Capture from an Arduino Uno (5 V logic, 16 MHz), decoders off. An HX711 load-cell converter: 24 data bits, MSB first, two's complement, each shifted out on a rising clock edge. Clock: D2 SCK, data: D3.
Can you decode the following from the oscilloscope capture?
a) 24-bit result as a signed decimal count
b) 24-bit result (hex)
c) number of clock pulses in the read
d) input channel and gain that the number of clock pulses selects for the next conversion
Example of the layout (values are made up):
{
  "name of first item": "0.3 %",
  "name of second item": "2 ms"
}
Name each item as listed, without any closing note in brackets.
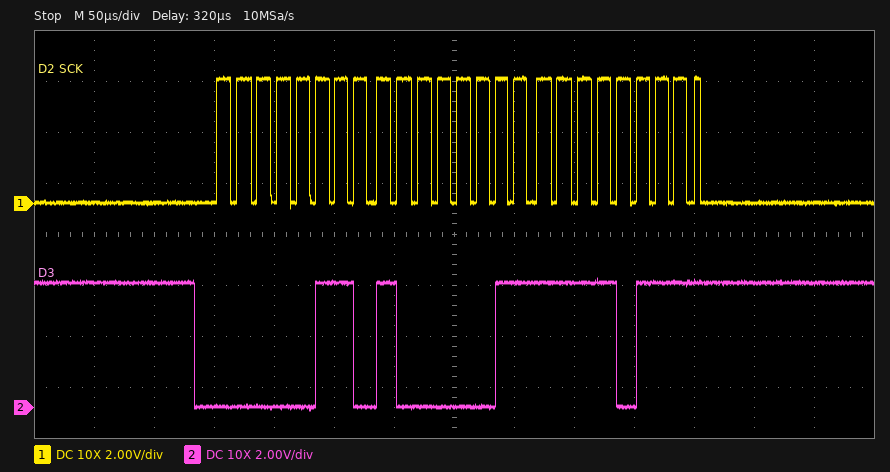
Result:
{
  "24-bit result as a signed decimal count": "426999",
  "24-bit result": "0x0683F7",
  "number of clock pulses in the read": "25",
  "input channel and gain that the number of clock pulses selects for the next conversion": "channel A, gain 128"
}
